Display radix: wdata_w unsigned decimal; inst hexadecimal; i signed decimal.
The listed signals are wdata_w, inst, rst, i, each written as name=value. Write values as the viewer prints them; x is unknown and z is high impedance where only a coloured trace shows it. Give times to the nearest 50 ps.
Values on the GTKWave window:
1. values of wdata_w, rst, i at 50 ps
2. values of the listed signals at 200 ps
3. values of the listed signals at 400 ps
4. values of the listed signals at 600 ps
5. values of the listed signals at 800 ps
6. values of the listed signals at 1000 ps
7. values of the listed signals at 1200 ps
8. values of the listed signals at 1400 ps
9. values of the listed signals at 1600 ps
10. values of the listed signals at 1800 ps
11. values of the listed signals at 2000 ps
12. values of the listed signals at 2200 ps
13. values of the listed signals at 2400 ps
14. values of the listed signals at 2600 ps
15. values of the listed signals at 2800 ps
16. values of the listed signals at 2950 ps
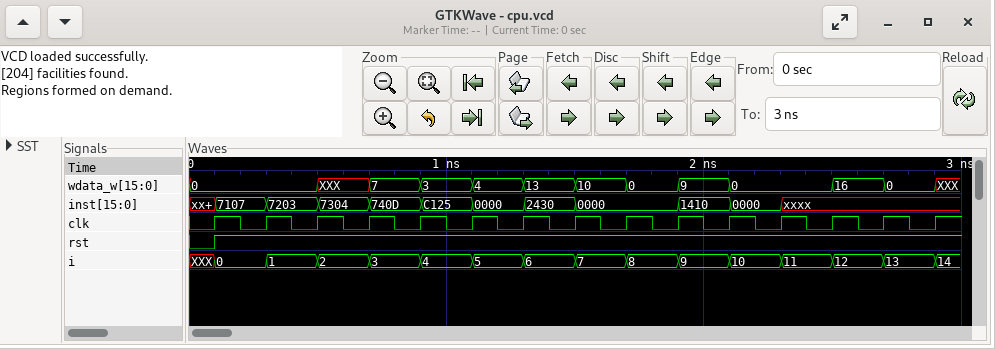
wdata_w=0, rst=0, i=XXX
wdata_w=0, inst=7107, rst=1, i=0
wdata_w=0, inst=7203, rst=1, i=1
wdata_w=XXX, inst=7304, rst=1, i=2
wdata_w=7, inst=740D, rst=1, i=3
wdata_w=3, inst=C125, rst=1, i=4
wdata_w=4, inst=0000, rst=1, i=5
wdata_w=13, inst=2430, rst=1, i=6
wdata_w=10, inst=0000, rst=1, i=7
wdata_w=0, inst=0000, rst=1, i=8
wdata_w=9, inst=1410, rst=1, i=9
wdata_w=0, inst=0000, rst=1, i=10
wdata_w=0, inst=xxxx, rst=1, i=11
wdata_w=16, inst=xxxx, rst=1, i=12
wdata_w=0, inst=xxxx, rst=1, i=13
wdata_w=XXX, inst=xxxx, rst=1, i=14
